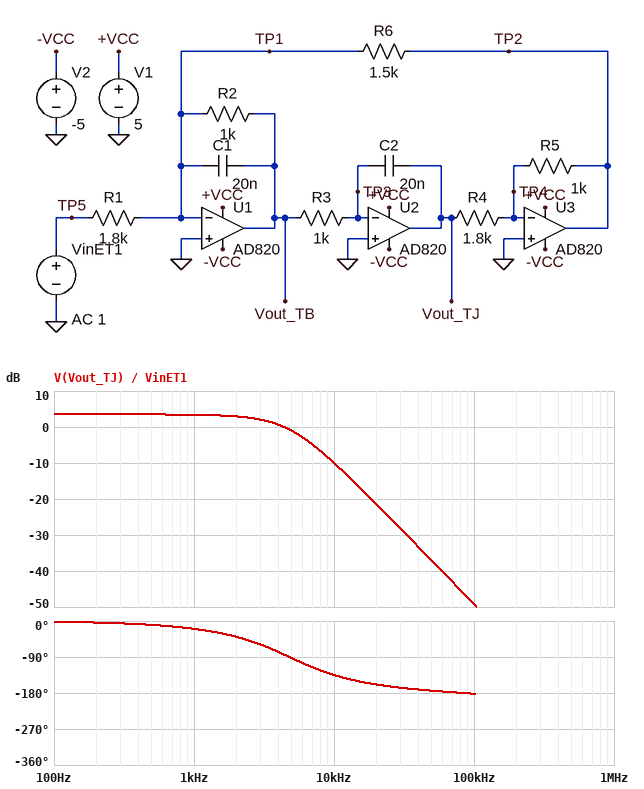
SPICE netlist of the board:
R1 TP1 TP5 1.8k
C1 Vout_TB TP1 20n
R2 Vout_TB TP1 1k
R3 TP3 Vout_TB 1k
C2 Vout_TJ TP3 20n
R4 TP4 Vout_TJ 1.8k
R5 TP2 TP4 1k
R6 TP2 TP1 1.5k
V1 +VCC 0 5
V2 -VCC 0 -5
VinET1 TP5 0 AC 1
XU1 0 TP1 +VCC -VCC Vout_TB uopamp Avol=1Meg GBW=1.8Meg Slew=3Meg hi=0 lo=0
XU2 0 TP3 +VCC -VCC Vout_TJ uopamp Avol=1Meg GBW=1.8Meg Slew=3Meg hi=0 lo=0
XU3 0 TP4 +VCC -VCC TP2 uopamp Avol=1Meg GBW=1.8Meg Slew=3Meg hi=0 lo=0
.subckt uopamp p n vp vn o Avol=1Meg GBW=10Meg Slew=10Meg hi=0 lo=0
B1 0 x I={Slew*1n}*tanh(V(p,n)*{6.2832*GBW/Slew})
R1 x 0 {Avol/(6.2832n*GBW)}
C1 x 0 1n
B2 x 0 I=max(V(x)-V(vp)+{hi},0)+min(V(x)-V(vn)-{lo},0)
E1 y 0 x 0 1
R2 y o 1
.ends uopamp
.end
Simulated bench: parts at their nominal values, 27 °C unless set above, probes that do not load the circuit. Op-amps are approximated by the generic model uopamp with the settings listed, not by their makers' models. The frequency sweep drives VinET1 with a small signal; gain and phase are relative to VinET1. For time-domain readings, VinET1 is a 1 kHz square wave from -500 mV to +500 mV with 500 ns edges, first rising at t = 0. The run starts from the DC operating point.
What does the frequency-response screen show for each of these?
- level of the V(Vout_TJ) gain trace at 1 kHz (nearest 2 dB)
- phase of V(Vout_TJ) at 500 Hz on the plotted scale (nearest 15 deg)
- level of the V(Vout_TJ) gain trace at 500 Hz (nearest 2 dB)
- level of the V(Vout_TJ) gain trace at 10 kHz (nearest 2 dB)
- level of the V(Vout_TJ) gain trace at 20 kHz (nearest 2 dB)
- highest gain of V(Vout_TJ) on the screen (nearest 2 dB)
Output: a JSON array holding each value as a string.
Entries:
["4 dB", "-15 deg", "4 dB", "-10 dB", "-22 dB", "4 dB"]
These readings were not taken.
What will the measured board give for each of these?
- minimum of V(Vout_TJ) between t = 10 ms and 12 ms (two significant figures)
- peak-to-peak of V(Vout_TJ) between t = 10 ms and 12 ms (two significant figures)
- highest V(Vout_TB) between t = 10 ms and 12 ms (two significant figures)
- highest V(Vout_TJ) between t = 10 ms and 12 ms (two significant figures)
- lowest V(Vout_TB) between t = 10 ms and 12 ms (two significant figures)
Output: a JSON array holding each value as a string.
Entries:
["-770 mV", "1.5 V", "380 mV", "770 mV", "-380 mV"]
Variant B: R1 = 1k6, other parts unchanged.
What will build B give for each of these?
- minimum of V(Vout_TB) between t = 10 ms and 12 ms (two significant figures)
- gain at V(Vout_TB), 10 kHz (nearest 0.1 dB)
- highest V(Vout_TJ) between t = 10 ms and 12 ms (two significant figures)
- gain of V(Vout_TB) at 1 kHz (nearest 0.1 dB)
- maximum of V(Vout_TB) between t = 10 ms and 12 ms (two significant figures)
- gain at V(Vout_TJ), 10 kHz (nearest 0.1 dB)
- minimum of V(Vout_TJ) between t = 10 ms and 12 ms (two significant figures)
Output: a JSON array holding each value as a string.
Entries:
["-430 mV", "-6.9 dB", "860 mV", "-13.6 dB", "430 mV", "-9.0 dB", "-860 mV"]
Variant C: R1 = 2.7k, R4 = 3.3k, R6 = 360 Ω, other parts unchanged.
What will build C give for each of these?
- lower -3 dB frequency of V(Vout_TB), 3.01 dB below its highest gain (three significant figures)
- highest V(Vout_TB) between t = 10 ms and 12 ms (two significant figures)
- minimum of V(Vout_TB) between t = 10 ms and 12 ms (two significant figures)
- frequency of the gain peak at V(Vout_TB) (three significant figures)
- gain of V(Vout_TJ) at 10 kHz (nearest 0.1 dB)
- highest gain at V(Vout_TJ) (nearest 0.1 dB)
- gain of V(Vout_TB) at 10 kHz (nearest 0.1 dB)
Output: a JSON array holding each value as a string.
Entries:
["4.33 kHz", "210 mV", "-210 mV", "7.23 kHz", "-11.9 dB", "-6.3 dB", "-9.9 dB"]
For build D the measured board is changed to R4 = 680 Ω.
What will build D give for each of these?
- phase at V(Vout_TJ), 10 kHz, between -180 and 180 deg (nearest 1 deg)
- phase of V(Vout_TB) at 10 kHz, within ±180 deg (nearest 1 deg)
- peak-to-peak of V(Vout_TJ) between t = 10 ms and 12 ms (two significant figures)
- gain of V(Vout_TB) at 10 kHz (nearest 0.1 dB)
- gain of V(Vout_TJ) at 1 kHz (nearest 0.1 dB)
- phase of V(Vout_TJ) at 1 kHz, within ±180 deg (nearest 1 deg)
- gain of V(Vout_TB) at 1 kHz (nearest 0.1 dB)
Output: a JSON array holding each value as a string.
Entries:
["-117 deg", "153 deg", "760 mV", "-5.9 dB", "-4.9 dB", "-7 deg", "-22.8 dB"]
